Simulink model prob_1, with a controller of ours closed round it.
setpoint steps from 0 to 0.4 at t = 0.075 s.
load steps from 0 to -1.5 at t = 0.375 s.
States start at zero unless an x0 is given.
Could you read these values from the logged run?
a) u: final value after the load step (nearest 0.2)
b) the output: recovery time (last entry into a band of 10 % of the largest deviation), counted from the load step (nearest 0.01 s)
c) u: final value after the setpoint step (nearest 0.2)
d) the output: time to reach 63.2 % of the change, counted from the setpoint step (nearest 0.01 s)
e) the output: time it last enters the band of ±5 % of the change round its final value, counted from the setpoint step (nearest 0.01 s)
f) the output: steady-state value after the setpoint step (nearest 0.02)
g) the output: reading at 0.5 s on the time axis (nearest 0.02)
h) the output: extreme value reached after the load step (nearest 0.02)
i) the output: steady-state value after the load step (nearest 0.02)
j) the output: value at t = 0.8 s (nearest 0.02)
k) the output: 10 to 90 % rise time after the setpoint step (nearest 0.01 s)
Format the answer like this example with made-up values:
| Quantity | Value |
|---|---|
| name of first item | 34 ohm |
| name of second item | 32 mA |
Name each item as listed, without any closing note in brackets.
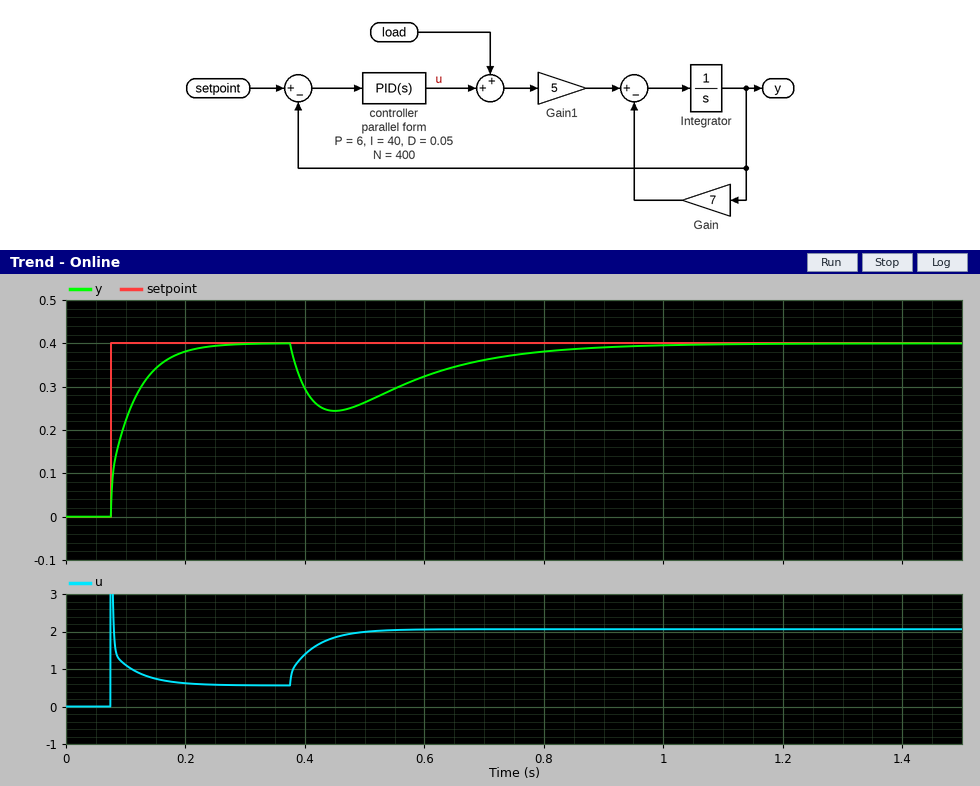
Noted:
| Quantity | Value |
|---|---|
| u: final value after the load step | 2.0 |
| the output: recovery time (last entry into a band of 10 % of the largest deviation), counted from the load step | 0.45 s |
| u: final value after the setpoint step | 0.6 |
| the output: time to reach 63.2 % of the change, counted from the setpoint step | 0.03 s |
| the output: time it last enters the band of ±5 % of the change round its final value, counted from the setpoint step | 0.12 s |
| the output: steady-state value after the setpoint step | 0.40 |
| the output: reading at 0.5 s on the time axis | 0.26 |
| the output: extreme value reached after the load step | 0.24 |
| the output: steady-state value after the load step | 0.40 |
| the output: value at t = 0.8 s | 0.38 |
| the output: 10 to 90 % rise time after the setpoint step | 0.09 s |
